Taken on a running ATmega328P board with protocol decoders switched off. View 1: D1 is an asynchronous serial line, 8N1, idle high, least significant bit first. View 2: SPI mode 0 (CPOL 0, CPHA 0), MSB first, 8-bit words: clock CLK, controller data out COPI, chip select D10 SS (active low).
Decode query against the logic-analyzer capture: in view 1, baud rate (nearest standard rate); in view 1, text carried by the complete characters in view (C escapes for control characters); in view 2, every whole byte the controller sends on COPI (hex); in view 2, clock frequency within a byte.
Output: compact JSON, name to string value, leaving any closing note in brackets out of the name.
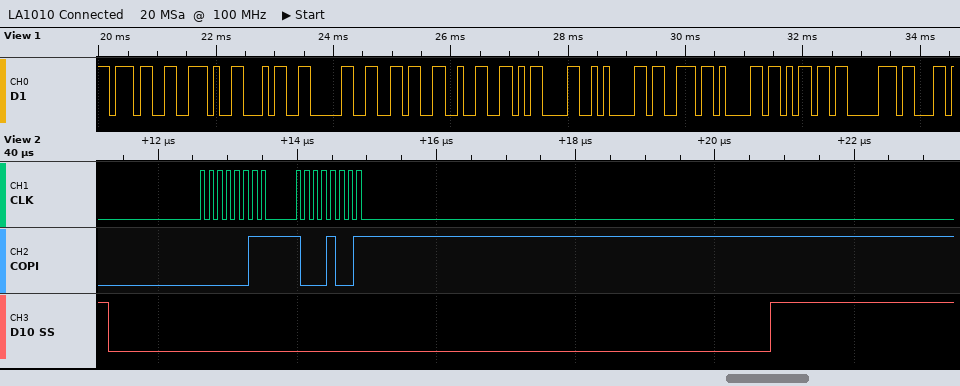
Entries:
{"in view 1, baud rate": "9600 baud", "in view 1, text carried by the complete characters in view": "\"7.4062\\r\\nsamp\"", "in view 2, every whole byte the controller sends on COPI": "03 89", "in view 2, clock frequency within a byte": "8 MHz"}
